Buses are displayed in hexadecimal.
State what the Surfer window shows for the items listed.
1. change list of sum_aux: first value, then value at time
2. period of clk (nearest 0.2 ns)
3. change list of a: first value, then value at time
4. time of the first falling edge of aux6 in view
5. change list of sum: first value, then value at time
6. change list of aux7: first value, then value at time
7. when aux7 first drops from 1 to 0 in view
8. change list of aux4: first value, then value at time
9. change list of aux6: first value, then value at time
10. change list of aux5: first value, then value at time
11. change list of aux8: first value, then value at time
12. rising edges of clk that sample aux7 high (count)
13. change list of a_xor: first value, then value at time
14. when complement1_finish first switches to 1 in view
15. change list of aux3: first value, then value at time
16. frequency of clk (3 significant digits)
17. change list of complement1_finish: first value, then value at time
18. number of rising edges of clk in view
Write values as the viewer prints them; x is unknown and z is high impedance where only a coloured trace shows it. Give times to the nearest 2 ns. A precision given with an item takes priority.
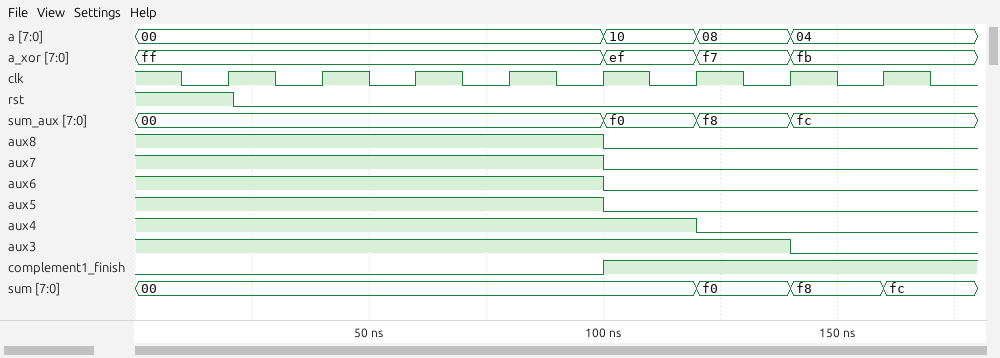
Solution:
00, f0 at 100 ns, f8 at 120 ns, fc at 140 ns
20 ns
00, 10 at 100 ns, 08 at 120 ns, 04 at 140 ns
100 ns
00, f0 at 120 ns, f8 at 140 ns, fc at 160 ns
1, 0 at 100 ns
100 ns
1, 0 at 120 ns
1, 0 at 100 ns
1, 0 at 100 ns
1, 0 at 100 ns
5
ff, ef at 100 ns, f7 at 120 ns, fb at 140 ns
100 ns
1, 0 at 140 ns
50.0 MHz
0, 1 at 100 ns
8
